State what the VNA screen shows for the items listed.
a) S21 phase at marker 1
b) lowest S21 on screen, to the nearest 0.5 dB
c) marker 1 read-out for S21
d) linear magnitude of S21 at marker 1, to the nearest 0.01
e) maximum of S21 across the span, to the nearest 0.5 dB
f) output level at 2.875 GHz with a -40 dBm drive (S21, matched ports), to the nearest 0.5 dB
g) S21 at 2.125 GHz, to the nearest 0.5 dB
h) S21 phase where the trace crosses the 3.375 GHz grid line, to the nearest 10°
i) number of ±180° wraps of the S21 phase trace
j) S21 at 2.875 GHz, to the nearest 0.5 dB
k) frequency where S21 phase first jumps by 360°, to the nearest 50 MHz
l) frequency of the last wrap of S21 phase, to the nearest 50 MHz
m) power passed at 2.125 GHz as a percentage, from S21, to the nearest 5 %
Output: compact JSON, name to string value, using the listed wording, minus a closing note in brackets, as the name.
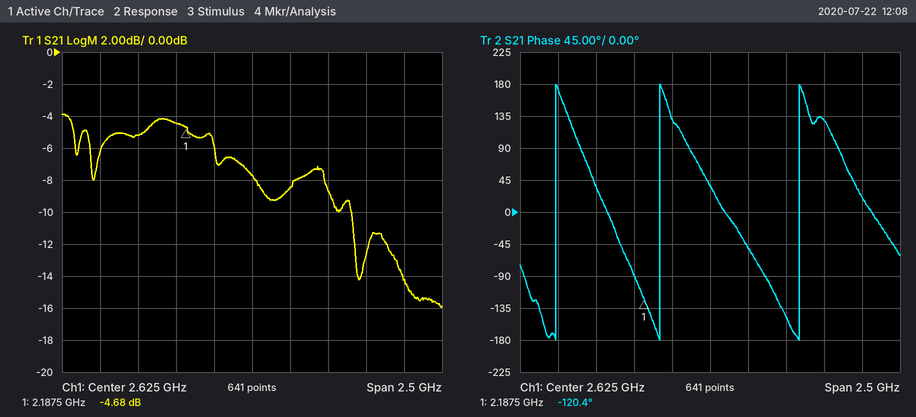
{"S21 phase at marker 1": "-120.4°", "lowest S21 on screen, to the nearest 0.5 dB": "-16.0 dB", "marker 1 read-out for S21": "-4.68 dB", "linear magnitude of S21 at marker 1, to the nearest 0.01": "0.58", "maximum of S21 across the span, to the nearest 0.5 dB": "-4.0 dB", "output level at 2.875 GHz with a -40 dBm drive (S21, matched ports), to the nearest 0.5 dB": "-48.5 dBm", "S21 at 2.125 GHz, to the nearest 0.5 dB": "-4.5 dB", "S21 phase where the trace crosses the 3.375 GHz grid line, to the nearest 10°": "130°", "number of ±180° wraps of the S21 phase trace": "3", "S21 at 2.875 GHz, to the nearest 0.5 dB": "-8.5 dB", "frequency where S21 phase first jumps by 360°, to the nearest 50 MHz": "1.60 GHz", "frequency of the last wrap of S21 phase, to the nearest 50 MHz": "3.20 GHz", "power passed at 2.125 GHz as a percentage, from S21, to the nearest 5 %": "35 %"}
